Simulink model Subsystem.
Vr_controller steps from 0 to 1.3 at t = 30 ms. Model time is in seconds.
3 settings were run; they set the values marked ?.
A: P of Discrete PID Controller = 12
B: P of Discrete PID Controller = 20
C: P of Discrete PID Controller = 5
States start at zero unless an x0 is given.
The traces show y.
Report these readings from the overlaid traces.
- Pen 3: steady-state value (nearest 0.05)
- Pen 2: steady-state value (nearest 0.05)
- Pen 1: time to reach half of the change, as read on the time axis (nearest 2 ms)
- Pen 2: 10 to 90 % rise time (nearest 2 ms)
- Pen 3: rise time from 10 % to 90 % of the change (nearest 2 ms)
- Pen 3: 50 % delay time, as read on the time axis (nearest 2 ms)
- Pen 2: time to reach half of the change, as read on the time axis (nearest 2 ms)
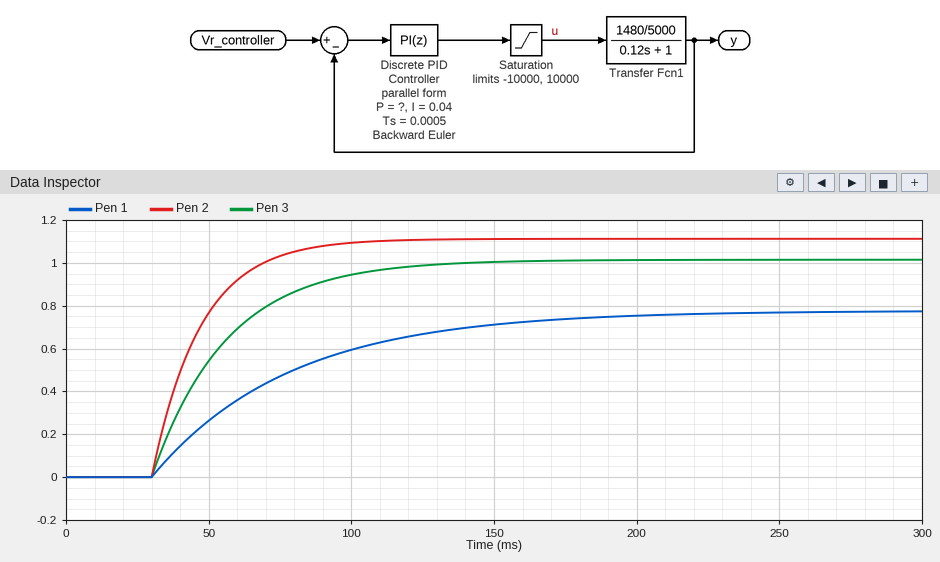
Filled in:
1.00
1.10
64 ms
38 ms
58 ms
48 ms
42 ms
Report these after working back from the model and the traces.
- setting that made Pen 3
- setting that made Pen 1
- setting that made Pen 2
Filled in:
A
C
B
